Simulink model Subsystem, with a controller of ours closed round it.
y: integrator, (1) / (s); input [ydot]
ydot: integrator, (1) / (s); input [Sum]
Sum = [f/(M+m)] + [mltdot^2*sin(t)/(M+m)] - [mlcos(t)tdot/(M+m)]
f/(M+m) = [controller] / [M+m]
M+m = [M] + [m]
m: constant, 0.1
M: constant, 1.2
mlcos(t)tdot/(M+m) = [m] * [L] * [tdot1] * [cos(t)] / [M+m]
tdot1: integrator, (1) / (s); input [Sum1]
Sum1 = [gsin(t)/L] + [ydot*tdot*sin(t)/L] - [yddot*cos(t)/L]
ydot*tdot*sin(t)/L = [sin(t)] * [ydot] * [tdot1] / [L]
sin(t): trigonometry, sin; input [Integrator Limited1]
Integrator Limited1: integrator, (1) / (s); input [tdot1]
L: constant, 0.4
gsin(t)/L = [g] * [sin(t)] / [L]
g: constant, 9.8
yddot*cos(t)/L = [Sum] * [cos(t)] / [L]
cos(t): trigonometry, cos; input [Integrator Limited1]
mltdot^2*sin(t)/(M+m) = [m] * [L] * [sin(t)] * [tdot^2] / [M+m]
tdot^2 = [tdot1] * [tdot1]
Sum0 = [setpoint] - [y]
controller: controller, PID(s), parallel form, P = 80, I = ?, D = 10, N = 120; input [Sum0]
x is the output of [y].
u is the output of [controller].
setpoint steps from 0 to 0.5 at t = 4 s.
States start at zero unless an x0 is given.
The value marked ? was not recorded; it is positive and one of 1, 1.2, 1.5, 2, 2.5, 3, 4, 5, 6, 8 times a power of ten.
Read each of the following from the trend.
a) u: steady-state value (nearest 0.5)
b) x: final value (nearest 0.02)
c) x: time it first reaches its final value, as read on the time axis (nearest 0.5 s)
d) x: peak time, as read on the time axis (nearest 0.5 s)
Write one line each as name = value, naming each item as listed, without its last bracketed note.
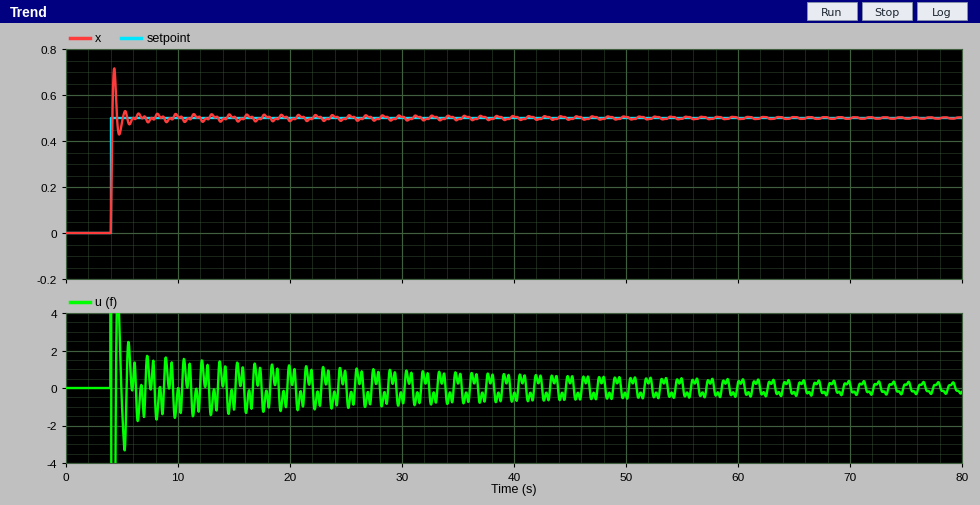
u: steady-state value = 0.0
x: final value = 0.50
x: time it first reaches its final value, as read on the time axis = 4.0 s
x: peak time, as read on the time axis = 4.5 s
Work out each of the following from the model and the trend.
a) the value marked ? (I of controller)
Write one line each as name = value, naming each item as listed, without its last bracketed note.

the value marked ? = 200
